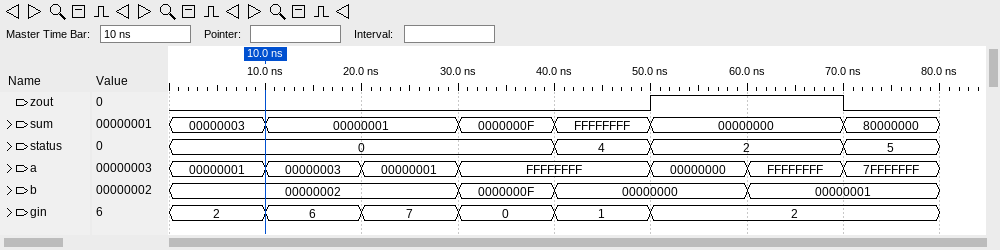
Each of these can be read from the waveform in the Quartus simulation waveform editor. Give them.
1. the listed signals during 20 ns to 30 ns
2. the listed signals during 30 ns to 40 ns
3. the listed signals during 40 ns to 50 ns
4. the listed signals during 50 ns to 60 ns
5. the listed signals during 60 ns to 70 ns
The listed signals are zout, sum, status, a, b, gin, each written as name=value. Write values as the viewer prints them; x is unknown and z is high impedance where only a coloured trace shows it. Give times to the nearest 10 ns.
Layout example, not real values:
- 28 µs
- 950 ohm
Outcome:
- zout=0, sum=00000001, status=0, a=00000001, b=00000002, gin=7
- zout=0, sum=0000000F, status=0, a=FFFFFFFF, b=0000000F, gin=0
- zout=0, sum=FFFFFFFF, status=4, a=FFFFFFFF, b=00000000, gin=1
- zout=1, sum=00000000, status=2, a=00000000, b=00000000, gin=2
- zout=1, sum=00000000, status=2, a=FFFFFFFF, b=00000001, gin=2
